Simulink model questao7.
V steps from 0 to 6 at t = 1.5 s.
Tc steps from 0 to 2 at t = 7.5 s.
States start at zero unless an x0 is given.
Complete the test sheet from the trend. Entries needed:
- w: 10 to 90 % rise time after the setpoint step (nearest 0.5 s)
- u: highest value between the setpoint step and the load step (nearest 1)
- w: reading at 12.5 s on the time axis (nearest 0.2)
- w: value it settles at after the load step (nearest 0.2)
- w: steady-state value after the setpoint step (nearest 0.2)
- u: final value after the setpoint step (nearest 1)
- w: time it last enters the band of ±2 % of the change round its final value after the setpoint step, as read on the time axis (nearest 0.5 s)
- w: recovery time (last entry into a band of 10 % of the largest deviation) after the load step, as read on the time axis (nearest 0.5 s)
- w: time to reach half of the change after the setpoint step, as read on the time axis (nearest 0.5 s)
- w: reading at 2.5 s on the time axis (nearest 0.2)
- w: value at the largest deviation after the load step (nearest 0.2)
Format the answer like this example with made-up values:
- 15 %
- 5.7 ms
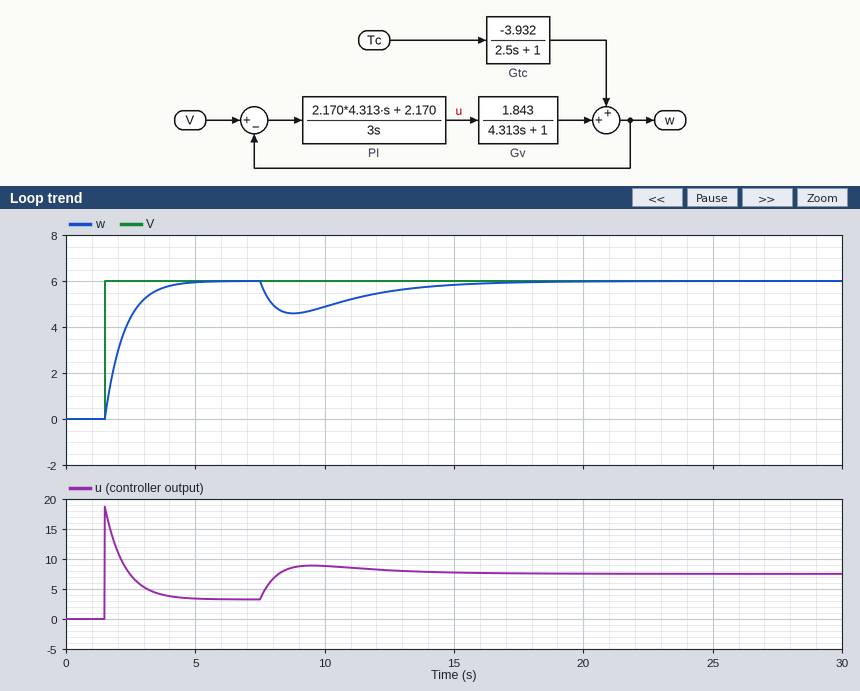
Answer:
- 1.5 s
- 19
- 5.6
- 6.0
- 6.0
- 3
- 4.5 s
- 15.5 s
- 2.0 s
- 4.4
- 4.6
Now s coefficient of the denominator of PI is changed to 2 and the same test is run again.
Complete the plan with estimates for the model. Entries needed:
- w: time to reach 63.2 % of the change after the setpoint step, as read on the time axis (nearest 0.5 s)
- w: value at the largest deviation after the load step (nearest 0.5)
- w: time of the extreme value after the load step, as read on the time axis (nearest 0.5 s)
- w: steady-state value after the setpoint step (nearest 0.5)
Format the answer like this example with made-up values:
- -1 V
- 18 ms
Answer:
- 2.0 s
- 5.0
- 8.5 s
- 6.0
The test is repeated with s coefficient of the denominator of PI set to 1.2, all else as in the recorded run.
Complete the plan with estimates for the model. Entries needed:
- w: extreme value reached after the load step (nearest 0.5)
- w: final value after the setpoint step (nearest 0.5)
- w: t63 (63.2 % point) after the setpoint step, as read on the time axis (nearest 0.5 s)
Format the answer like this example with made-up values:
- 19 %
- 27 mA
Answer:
- 5.5
- 6.0
- 2.0 s
